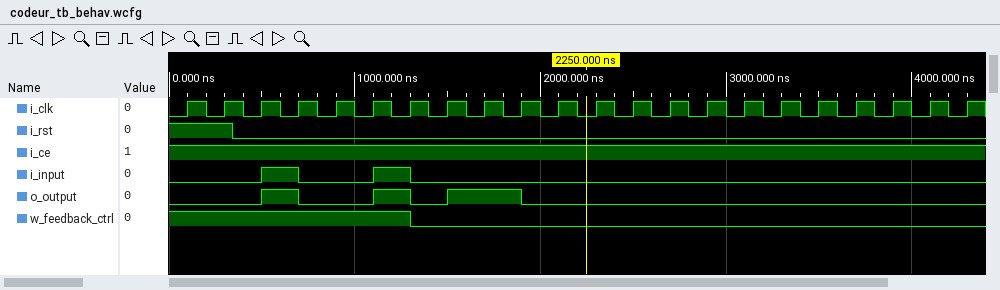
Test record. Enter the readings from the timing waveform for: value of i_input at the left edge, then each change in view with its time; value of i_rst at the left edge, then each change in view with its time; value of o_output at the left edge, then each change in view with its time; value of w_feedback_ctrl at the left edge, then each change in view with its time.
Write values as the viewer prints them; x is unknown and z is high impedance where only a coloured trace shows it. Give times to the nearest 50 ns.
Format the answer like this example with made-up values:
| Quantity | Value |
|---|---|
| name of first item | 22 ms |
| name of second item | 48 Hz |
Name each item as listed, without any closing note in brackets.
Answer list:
| Quantity | Value |
|---|---|
| value of i_input at the left edge, then each change in view with its time | 0, 1 at 500 ns, 0 at 700 ns, 1 at 1100 ns, 0 at 1300 ns |
| value of i_rst at the left edge, then each change in view with its time | 1, 0 at 350 ns |
| value of o_output at the left edge, then each change in view with its time | 0, 1 at 500 ns, 0 at 700 ns, 1 at 1100 ns, 0 at 1300 ns, 1 at 1500 ns, 0 at 1900 ns |
| value of w_feedback_ctrl at the left edge, then each change in view with its time | 1, 0 at 1300 ns |
